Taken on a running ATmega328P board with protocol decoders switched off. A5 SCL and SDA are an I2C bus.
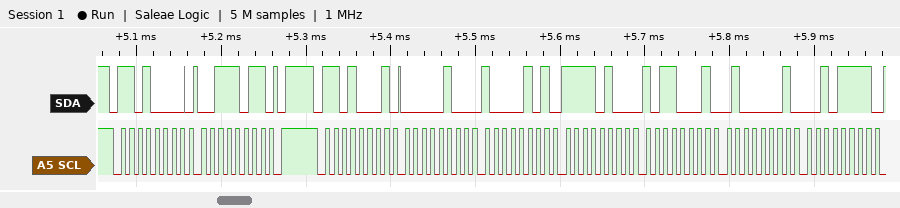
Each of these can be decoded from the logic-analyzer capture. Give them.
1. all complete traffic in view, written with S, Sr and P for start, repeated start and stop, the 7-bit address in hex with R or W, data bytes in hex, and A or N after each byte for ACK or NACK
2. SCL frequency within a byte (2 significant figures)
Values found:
S 68W A 3B A P S 68R A 04 A 85 A F4 A B1 A 41 A 2F A
100 kHz
